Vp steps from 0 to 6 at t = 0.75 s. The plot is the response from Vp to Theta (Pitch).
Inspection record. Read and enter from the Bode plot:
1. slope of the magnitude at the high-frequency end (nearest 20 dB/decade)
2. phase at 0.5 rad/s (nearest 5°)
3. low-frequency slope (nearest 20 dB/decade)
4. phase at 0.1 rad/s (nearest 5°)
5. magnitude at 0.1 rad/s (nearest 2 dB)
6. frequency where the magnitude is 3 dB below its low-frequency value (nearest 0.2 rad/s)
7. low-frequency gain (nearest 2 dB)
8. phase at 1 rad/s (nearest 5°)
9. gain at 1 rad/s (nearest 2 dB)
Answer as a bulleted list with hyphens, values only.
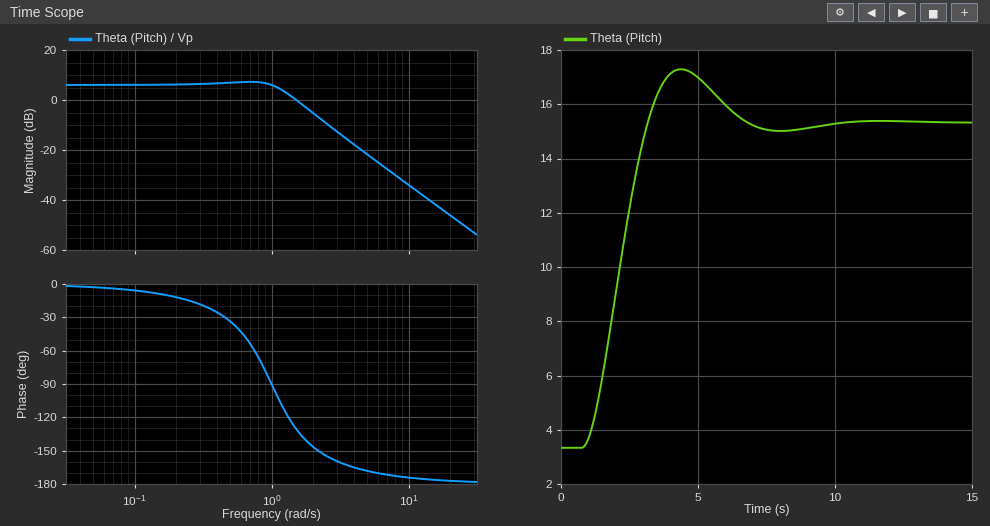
- -40 dB/decade
- -35°
- 0 dB/decade
- -5°
- 6 dB
- 1.2 rad/s
- 6 dB
- -90°
- 6 dB
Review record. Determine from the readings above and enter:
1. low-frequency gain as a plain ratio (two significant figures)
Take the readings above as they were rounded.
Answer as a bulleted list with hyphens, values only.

- 2.0
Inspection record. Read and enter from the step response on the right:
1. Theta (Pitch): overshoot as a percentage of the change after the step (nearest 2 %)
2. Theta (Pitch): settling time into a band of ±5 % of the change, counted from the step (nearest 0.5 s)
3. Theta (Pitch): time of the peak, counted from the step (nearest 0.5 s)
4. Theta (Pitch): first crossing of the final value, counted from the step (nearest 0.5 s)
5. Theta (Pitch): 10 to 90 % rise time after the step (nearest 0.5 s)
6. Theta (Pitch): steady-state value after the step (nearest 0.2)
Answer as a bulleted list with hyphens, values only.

- 16 %
- 5.5 s
- 3.5 s
- 2.5 s
- 1.5 s
- 15.4
